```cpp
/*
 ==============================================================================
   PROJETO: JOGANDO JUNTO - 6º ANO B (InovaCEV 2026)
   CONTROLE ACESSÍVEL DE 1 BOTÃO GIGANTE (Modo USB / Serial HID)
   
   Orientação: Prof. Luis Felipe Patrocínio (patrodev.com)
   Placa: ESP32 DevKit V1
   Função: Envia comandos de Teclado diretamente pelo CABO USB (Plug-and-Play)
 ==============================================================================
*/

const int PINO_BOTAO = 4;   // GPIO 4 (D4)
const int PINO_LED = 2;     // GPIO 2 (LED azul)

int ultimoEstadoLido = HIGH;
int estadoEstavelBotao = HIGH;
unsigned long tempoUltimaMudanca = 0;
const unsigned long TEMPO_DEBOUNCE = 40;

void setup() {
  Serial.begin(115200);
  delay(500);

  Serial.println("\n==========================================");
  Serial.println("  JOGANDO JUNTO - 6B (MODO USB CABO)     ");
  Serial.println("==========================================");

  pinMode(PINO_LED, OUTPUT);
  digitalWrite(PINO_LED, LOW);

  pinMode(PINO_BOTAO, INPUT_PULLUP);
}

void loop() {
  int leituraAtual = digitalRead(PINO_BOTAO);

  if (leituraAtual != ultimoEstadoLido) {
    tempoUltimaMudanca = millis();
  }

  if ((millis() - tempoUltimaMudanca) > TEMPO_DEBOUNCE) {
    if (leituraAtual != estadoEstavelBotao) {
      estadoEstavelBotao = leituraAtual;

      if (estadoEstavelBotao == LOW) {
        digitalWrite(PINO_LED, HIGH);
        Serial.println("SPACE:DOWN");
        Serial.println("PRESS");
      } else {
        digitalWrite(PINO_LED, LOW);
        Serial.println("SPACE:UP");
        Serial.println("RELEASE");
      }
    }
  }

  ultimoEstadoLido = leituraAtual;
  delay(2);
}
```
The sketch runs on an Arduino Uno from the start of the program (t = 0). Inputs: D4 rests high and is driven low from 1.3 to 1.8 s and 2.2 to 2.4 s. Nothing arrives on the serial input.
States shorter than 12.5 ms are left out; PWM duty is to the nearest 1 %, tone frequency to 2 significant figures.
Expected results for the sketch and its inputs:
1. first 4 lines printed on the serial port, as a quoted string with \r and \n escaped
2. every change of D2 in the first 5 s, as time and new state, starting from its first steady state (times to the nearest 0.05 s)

"\n==========================================\r\n  JOGANDO JUNTO - 6B (MODO USB CABO)     \r\n==========================================\r\n"
0.5 s low; 1.35 s high; 1.85 s low; 2.25 s high; 2.45 s low
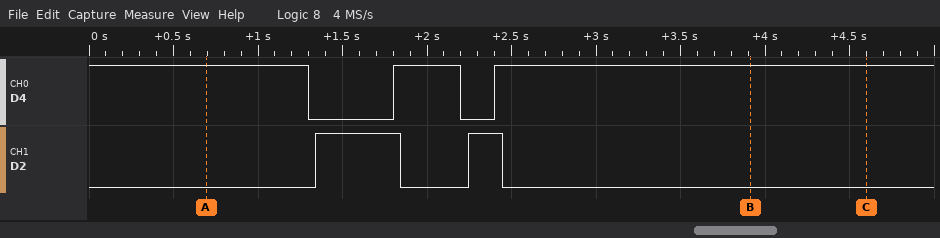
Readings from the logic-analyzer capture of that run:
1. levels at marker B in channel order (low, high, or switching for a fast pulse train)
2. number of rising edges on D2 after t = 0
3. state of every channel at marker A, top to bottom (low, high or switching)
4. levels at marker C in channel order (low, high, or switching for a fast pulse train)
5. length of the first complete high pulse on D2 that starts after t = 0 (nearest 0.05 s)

D4 high, D2 low
2
D4 high, D2 low
D4 high, D2 low
0.50 s
